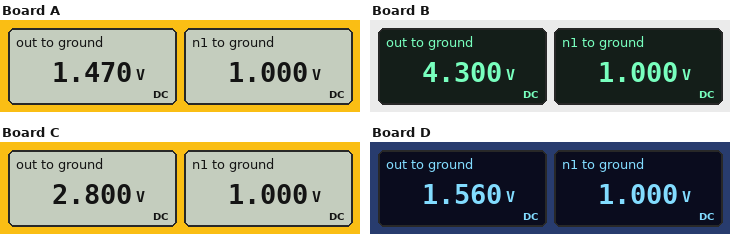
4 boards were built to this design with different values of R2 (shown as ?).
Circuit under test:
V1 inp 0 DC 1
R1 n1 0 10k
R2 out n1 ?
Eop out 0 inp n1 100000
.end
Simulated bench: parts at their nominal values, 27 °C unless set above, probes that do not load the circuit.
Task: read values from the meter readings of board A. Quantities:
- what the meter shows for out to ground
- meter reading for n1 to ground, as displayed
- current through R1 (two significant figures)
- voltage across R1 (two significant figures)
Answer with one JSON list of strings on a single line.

["1.470 V", "1.000 V", "100 µA", "1.0 V"]
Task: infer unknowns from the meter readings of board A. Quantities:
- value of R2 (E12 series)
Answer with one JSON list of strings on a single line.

["4.7 kΩ"]
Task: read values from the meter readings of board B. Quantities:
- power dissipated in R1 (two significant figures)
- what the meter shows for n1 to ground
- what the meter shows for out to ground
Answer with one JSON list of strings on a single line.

["100 µW", "1.000 V", "4.300 V"]
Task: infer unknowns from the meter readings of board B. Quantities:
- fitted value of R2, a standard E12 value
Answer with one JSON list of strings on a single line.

["33 kΩ"]
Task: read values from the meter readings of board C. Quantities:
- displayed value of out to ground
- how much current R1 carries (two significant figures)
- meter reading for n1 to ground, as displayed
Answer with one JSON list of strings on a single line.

["2.800 V", "100 µA", "1.000 V"]
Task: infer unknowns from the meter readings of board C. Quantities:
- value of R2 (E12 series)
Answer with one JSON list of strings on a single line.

["18 kΩ"]
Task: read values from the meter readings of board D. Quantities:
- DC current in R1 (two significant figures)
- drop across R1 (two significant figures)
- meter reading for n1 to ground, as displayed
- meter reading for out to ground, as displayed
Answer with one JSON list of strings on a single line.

["100 µA", "1.0 V", "1.000 V", "1.560 V"]
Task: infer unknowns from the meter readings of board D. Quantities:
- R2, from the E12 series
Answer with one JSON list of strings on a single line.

["5.6 kΩ"]
